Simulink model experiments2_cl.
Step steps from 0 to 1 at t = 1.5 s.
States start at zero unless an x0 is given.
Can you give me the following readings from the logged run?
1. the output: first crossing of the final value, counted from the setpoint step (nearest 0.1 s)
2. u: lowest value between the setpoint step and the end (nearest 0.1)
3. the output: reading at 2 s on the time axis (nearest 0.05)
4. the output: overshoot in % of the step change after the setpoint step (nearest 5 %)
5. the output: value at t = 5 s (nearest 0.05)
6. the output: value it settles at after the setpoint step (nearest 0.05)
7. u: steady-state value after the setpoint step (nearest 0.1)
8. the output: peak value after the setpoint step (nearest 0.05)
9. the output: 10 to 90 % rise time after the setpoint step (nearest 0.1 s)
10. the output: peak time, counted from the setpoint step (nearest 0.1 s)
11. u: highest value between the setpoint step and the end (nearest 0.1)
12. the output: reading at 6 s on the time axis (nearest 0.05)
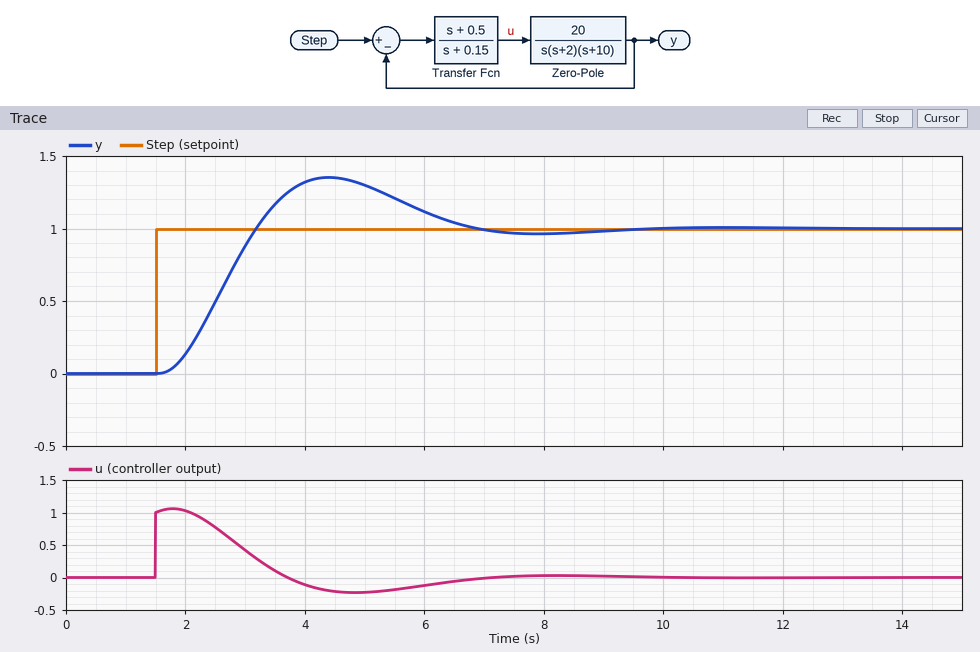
1.7 s
-0.2
0.15
35 %
1.30
1.00
0.0
1.35
1.1 s
2.9 s
1.1
1.10
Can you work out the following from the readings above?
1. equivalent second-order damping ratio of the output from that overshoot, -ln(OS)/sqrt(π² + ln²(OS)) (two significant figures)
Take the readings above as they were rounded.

0.32
